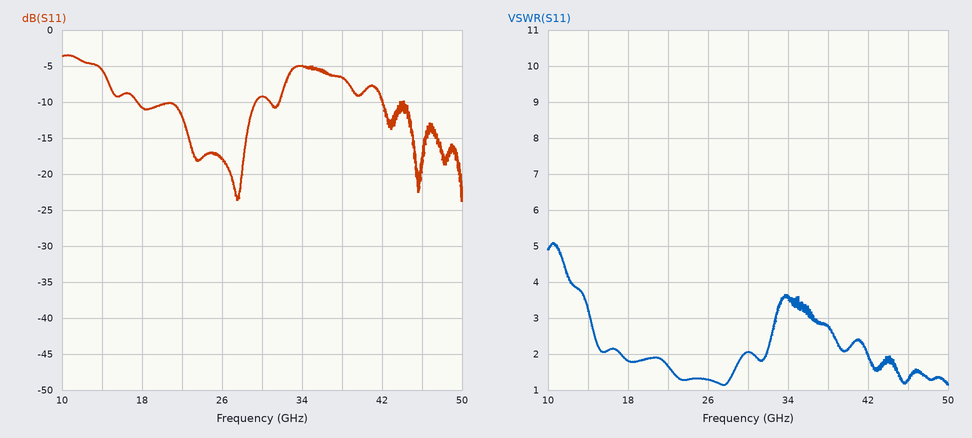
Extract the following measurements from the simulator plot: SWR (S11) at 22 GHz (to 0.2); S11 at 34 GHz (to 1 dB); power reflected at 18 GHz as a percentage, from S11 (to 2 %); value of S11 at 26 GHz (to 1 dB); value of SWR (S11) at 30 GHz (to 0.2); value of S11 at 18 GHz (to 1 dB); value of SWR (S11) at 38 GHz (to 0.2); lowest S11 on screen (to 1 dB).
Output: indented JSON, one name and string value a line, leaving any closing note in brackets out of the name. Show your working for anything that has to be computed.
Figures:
{
  "SWR (S11) at 22 GHz": "1.6",
  "S11 at 34 GHz": "-5 dB",
  "power reflected at 18 GHz as a percentage, from S11": "10^(-11/10) ≈ 8 %",
  "value of S11 at 26 GHz": "-18 dB",
  "value of SWR (S11) at 30 GHz": "2.0",
  "value of S11 at 18 GHz": "-11 dB",
  "value of SWR (S11) at 38 GHz": "2.8",
  "lowest S11 on screen": "-24 dB"
}
